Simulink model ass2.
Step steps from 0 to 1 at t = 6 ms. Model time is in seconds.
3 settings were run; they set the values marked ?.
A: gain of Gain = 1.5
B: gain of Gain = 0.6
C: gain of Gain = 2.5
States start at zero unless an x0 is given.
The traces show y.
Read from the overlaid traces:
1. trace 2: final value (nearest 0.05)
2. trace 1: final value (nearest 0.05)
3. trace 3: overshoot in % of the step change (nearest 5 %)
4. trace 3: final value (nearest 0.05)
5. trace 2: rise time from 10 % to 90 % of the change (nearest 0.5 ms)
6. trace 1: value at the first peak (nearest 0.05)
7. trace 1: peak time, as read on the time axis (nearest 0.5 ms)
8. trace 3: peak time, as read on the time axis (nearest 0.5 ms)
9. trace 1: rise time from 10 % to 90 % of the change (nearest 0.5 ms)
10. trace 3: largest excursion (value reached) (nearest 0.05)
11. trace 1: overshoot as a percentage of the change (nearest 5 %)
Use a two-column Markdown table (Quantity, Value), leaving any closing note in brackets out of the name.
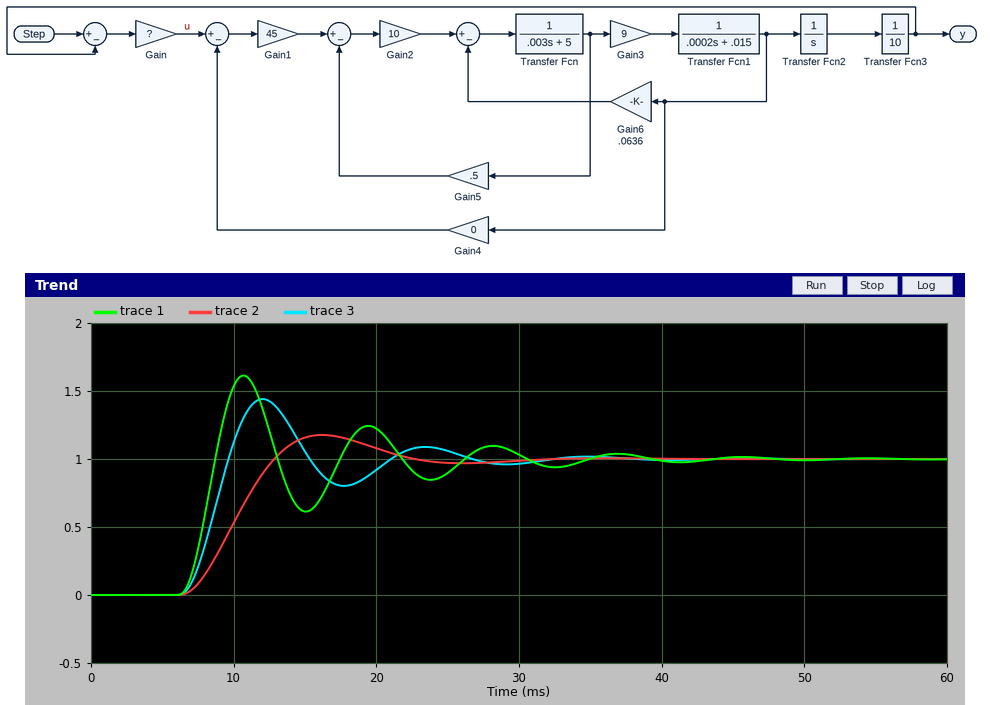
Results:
| Quantity | Value |
|---|---|
| trace 2: final value | 1.00 |
| trace 1: final value | 1.00 |
| trace 3: overshoot in % of the step change | 45 % |
| trace 3: final value | 1.00 |
| trace 2: rise time from 10 % to 90 % of the change | 4.5 ms |
| trace 1: value at the first peak | 1.60 |
| trace 1: peak time, as read on the time axis | 10.5 ms |
| trace 3: peak time, as read on the time axis | 12.0 ms |
| trace 1: rise time from 10 % to 90 % of the change | 1.5 ms |
| trace 3: largest excursion (value reached) | 1.45 |
| trace 1: overshoot as a percentage of the change | 60 % |
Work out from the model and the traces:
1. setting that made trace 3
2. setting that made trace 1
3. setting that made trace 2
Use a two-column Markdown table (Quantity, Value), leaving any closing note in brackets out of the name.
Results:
| Quantity | Value |
|---|---|
| setting that made trace 3 | A |
| setting that made trace 1 | C |
| setting that made trace 2 | B |
